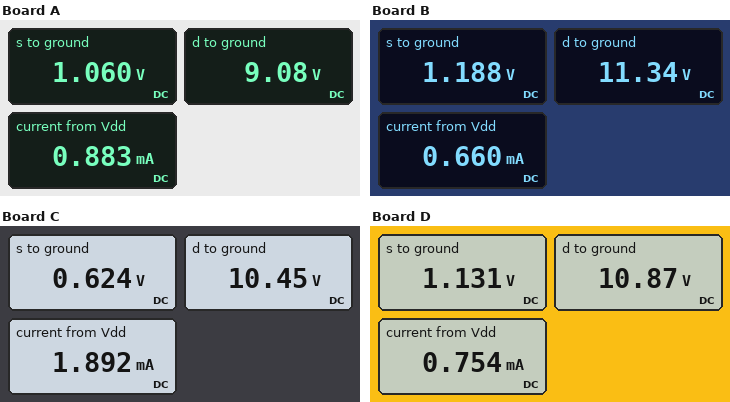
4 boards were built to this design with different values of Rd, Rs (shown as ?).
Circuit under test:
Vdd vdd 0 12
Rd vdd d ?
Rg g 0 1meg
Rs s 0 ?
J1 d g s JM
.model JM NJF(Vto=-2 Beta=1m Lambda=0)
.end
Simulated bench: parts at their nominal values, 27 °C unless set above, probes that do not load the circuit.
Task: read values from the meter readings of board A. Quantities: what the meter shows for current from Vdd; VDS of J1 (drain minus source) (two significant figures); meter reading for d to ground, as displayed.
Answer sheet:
0.883 mA
8.0 V
9.08 V
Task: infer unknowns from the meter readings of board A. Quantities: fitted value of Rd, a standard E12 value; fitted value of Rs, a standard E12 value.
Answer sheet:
3.3 kΩ
1.2 kΩ
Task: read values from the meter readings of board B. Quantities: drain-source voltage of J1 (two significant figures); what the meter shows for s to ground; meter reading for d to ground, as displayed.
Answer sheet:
10 V
1.188 V
11.34 V
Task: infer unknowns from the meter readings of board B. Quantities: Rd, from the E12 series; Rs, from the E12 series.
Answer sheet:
1 kΩ
1.8 kΩ
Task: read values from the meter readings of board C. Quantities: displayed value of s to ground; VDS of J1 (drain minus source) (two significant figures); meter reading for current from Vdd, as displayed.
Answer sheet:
0.624 V
9.8 V
1.892 mA
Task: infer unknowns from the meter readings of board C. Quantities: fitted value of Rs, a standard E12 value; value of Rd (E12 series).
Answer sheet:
330 Ω
820 Ω
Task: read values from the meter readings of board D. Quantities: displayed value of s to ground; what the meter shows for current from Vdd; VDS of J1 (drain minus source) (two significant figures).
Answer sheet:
1.131 V
0.754 mA
9.7 V
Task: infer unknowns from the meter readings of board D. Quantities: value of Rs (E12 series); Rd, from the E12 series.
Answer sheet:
1.5 kΩ
1.5 kΩ
